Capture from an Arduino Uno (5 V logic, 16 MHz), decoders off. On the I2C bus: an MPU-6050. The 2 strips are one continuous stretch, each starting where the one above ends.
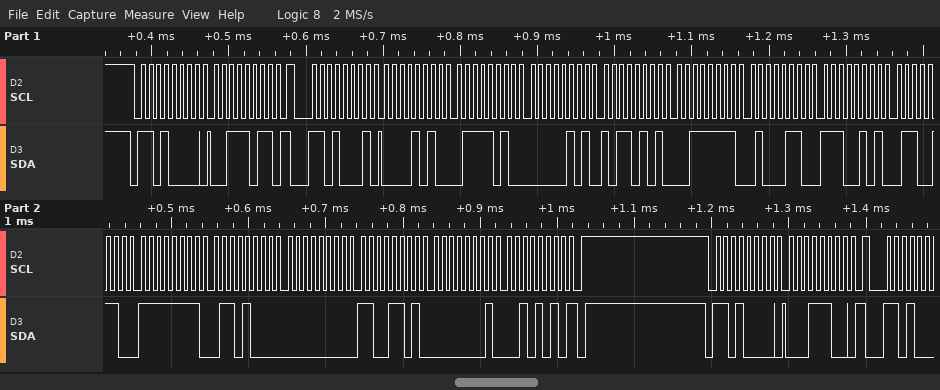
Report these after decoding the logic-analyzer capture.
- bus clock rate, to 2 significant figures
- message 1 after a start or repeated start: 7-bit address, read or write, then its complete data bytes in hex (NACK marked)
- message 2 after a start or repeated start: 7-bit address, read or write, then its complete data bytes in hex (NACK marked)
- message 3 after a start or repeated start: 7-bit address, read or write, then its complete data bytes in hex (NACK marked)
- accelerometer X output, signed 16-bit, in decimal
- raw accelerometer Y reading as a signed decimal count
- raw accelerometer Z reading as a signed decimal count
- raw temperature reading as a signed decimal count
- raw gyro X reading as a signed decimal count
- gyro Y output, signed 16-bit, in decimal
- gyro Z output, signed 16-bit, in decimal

100 kHz
0x68 write: 3B
0x68 read: 0A 7A 05 B5 3F 46 E5 66 FF 68 00 CD 01 2A NACK
0x68 write: 1C
2682
1461
16198
-6810
-152
205
298
